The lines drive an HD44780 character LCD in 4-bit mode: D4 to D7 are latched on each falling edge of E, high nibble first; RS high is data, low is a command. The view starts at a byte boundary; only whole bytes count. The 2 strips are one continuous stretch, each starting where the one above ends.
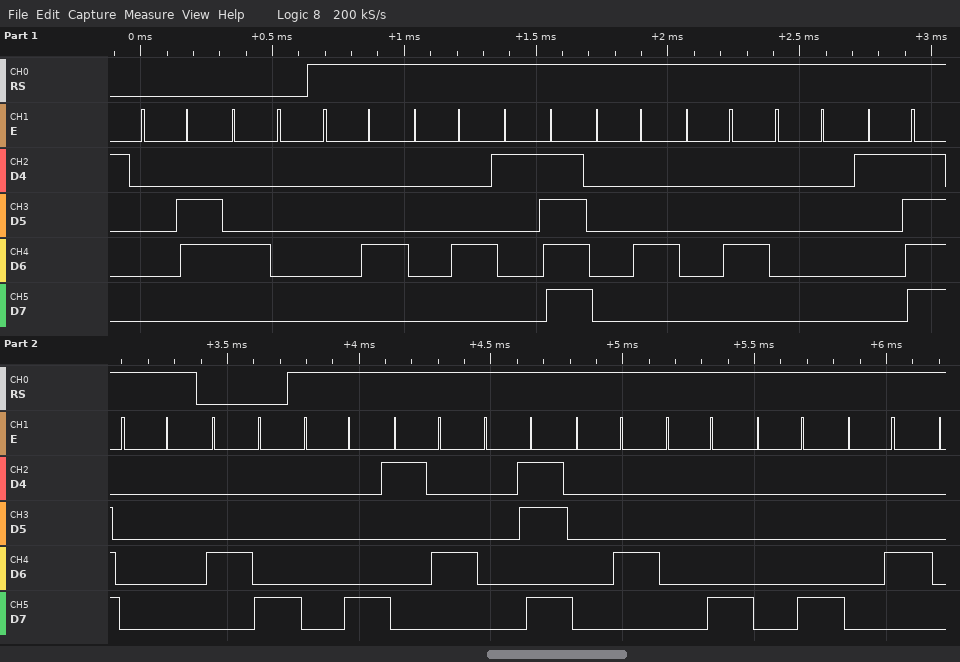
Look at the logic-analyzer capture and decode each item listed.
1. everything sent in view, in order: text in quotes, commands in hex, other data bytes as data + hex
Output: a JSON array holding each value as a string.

["0x06 0x40 data 04 04 1F 04 04 00 1F 00 0x48 data 08 14 0B 04 08 08 04"]
